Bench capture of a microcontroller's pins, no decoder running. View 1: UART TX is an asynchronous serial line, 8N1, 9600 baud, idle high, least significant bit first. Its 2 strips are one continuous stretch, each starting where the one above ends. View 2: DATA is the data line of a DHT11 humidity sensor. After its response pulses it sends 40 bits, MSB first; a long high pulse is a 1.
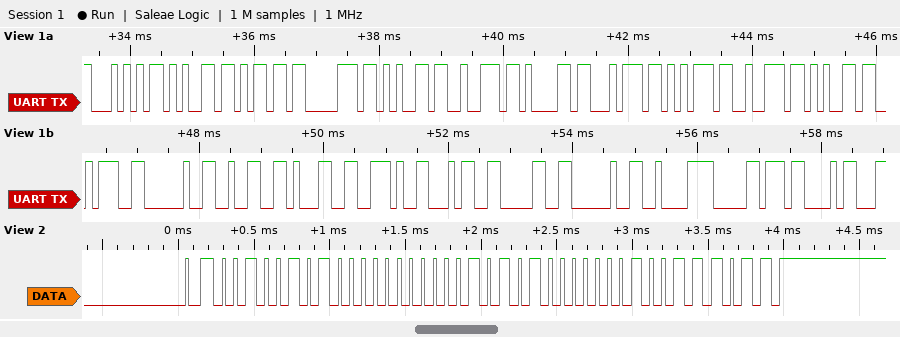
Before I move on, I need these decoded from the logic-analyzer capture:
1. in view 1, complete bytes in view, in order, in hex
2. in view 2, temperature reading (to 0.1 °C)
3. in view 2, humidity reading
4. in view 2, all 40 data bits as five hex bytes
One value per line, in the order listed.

0x54 0x65 0x6D 0x70 0x65 0x72 0x61 0x74 0x75 0x72 0x65 0x3A 0x20 0x32 0x31 0x2E 0x34 0x30 0x20 0xC2 0xB0 0x43
21.1 °C
37 %
25 00 15 01 3B
